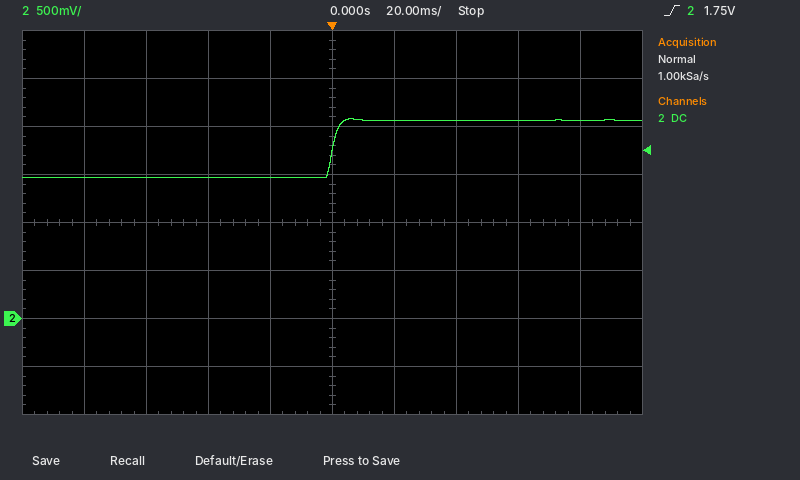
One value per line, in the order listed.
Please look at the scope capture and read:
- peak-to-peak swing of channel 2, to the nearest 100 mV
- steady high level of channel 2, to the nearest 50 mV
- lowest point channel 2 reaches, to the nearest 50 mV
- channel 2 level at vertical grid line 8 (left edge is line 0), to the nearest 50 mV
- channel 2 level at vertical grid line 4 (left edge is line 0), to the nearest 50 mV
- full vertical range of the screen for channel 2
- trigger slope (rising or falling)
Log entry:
600 mV
2.05 V
1.45 V
2.05 V
1.45 V
4 V
rising
